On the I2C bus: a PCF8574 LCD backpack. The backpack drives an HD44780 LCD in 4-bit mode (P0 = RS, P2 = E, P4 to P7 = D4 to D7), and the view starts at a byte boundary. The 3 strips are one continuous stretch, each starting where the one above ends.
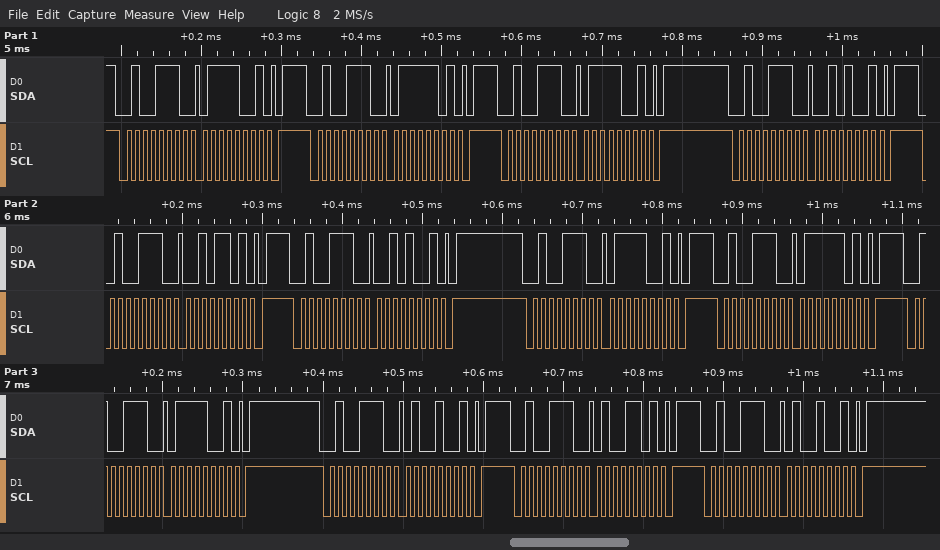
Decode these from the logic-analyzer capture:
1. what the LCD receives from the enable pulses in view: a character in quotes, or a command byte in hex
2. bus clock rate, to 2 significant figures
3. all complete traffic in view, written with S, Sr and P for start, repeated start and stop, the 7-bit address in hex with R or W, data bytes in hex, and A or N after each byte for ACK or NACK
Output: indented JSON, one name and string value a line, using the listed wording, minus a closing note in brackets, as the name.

{
  "what the LCD receives from the enable pulses in view: a character in quotes, or a command byte in hex": "'r' 't'",
  "bus clock rate, to 2 significant figures": "100 kHz",
  "all complete traffic in view, written with S, Sr and P for start, repeated start and stop, the 7-bit address in hex with R or W, data bytes in hex, and A or N after each byte for ACK or NACK": "S 27W A 79 A P S 27W A 7D A P S 27W A 79 A P S 27W A 29 A P S 27W A 2D A P S 27W A 29 A P S 27W A 79 A P S 27W A 7D A P S 27W A 79 A P S 27W A 49 A P S 27W A 4D A P S 27W A 49 A P"
}
